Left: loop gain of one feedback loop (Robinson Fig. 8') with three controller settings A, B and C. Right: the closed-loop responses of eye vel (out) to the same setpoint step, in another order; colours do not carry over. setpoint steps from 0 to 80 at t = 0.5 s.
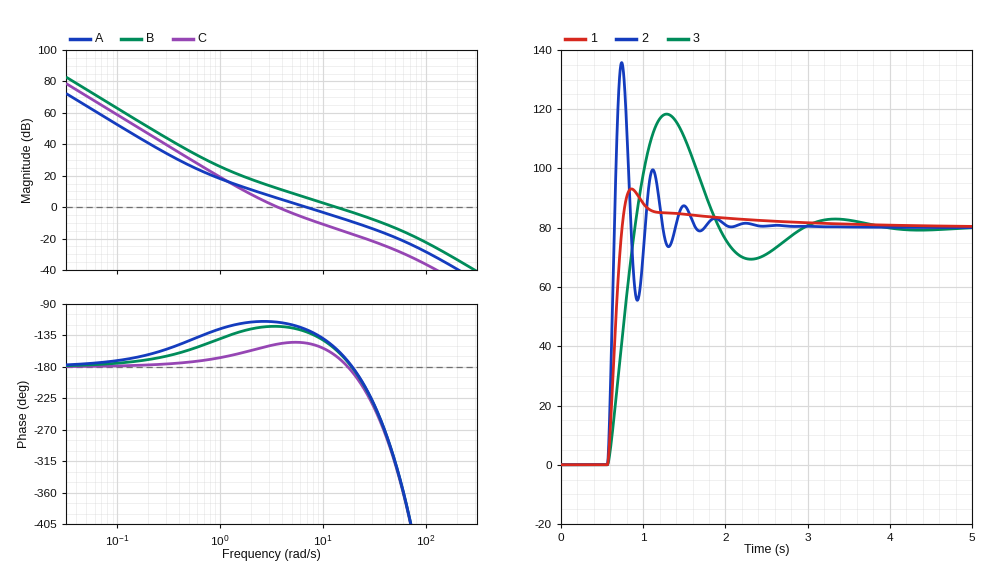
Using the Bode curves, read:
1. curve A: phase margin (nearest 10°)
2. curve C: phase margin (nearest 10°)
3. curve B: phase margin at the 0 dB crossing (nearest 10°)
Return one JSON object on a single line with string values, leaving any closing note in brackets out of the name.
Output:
{"curve A: phase margin": "50°", "curve C: phase margin": "30°", "curve B: phase margin at the 0 dB crossing": "20°"}
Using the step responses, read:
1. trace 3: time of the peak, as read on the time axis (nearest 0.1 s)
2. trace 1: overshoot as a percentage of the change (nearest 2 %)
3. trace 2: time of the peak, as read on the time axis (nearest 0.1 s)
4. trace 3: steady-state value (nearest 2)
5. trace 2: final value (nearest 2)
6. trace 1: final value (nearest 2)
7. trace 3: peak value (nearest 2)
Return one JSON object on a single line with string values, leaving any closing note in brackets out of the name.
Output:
{"trace 3: time of the peak, as read on the time axis": "1.3 s", "trace 1: overshoot as a percentage of the change": "16 %", "trace 2: time of the peak, as read on the time axis": "0.7 s", "trace 3: steady-state value": "80", "trace 2: final value": "80", "trace 1: final value": "80", "trace 3: peak value": "118"}
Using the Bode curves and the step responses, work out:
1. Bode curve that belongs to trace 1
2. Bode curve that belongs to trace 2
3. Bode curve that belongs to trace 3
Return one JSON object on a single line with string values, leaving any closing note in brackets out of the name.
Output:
{"Bode curve that belongs to trace 1": "A", "Bode curve that belongs to trace 2": "B", "Bode curve that belongs to trace 3": "C"}
